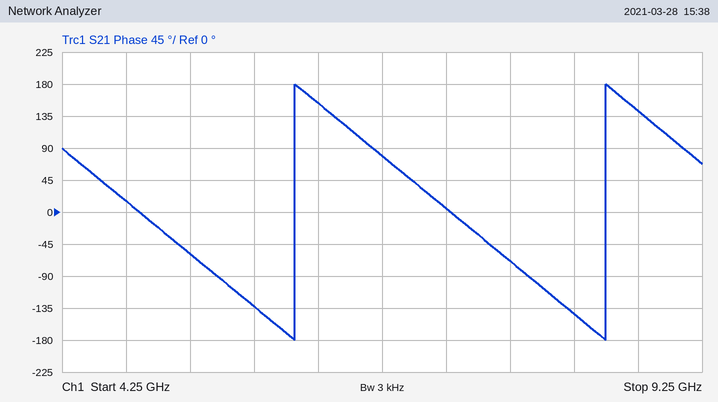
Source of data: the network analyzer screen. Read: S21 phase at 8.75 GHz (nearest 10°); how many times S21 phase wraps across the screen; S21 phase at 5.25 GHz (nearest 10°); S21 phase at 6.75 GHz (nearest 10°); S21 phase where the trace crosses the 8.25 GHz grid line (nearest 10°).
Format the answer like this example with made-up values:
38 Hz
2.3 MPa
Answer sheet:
140°
2
-60°
80°
-140°
